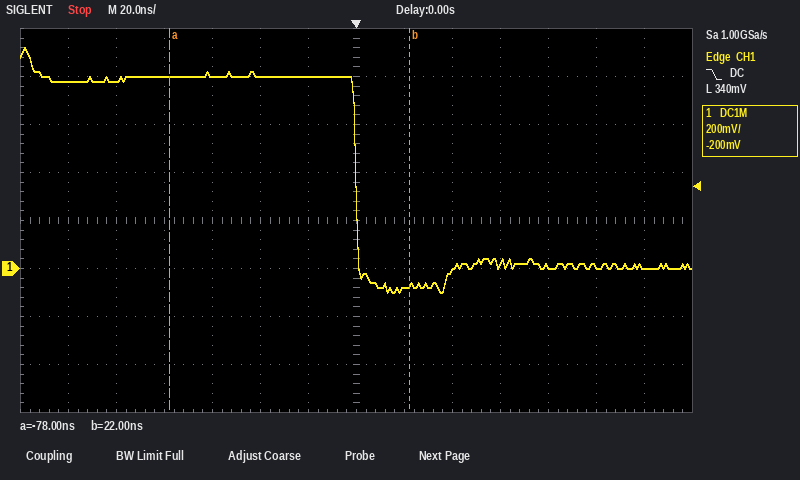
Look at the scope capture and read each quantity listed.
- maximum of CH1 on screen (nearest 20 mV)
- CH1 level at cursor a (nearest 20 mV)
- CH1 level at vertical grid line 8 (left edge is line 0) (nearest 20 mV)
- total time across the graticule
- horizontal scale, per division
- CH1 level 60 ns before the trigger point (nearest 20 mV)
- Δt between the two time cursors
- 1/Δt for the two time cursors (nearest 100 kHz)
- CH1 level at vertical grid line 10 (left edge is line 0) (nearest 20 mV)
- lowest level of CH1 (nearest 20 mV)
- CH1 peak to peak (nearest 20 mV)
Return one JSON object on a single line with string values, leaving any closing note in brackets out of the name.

{"maximum of CH1 on screen": "920 mV", "CH1 level at cursor a": "800 mV", "CH1 level at vertical grid line 8 (left edge is line 0)": "-80 mV", "total time across the graticule": "280 ns", "horizontal scale, per division": "20 ns", "CH1 level 60 ns before the trigger point": "800 mV", "Δt between the two time cursors": "100 ns", "1/Δt for the two time cursors": "10.0 MHz", "CH1 level at vertical grid line 10 (left edge is line 0)": "20 mV", "lowest level of CH1": "-100 mV", "CH1 peak to peak": "1.02 V"}
